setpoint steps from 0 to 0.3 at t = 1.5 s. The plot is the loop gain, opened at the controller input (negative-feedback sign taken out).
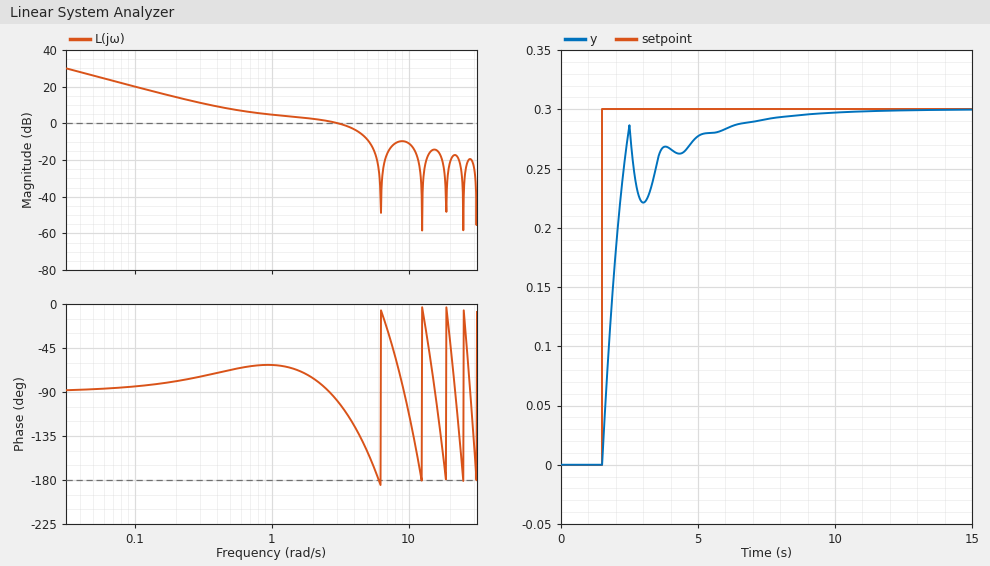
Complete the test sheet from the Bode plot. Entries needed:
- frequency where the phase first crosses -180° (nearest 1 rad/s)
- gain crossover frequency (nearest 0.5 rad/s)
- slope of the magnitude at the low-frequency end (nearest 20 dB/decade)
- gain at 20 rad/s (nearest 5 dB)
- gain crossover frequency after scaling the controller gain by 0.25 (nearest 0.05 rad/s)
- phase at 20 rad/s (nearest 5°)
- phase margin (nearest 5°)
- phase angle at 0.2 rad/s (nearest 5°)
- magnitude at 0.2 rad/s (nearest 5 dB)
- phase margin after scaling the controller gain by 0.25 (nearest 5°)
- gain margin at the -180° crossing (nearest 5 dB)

6 rad/s
3.0 rad/s
-20 dB/decade
-20 dB
0.25 rad/s
-35°
80°
-80°
15 dB
105°
25 dB
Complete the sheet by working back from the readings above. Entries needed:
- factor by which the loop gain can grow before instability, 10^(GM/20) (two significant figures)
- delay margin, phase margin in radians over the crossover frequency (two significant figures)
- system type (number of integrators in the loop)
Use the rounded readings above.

18
0.47 s
1
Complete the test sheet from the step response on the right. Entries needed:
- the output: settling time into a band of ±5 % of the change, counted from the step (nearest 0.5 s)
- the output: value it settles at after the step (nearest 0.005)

4.5 s
0.300
